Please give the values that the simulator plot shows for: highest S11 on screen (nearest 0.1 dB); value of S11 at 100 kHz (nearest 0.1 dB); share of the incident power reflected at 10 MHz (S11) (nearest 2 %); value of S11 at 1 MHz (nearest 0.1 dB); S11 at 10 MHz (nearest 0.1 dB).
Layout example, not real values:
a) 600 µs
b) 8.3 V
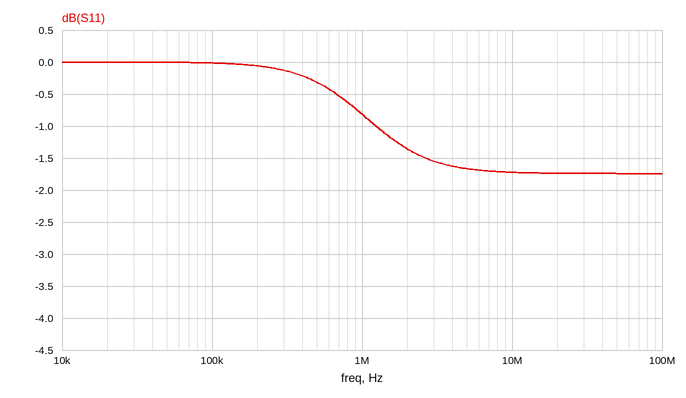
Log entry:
a) 0.0 dB
b) 0.0 dB
c) 68 %
d) -0.8 dB
e) -1.7 dB
